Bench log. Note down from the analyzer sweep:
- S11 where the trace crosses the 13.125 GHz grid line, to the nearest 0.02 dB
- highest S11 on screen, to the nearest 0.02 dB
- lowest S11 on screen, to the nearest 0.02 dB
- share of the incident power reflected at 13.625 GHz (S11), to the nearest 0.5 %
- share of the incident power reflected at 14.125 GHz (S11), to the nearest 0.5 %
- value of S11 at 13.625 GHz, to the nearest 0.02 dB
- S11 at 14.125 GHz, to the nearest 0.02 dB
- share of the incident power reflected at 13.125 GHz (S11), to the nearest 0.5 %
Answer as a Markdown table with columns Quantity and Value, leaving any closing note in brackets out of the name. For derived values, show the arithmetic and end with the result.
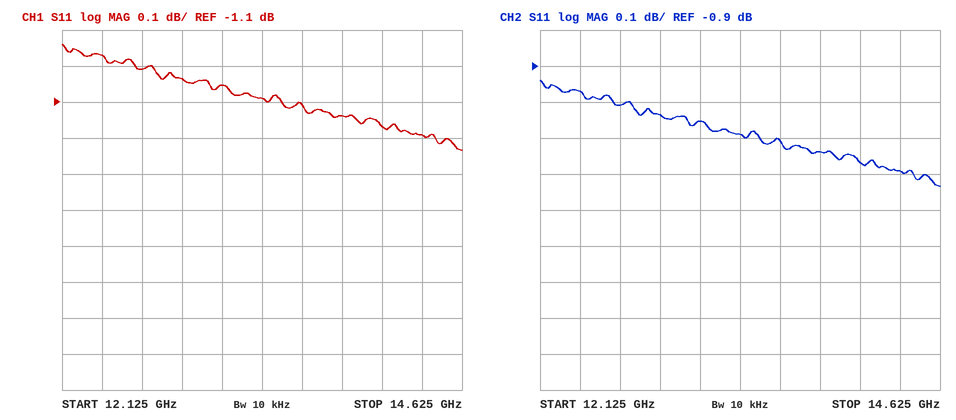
| Quantity | Value |
|---|---|
| S11 where the trace crosses the 13.125 GHz grid line, to the nearest 0.02 dB | -1.06 dB |
| highest S11 on screen, to the nearest 0.02 dB | -0.94 dB |
| lowest S11 on screen, to the nearest 0.02 dB | -1.24 dB |
| share of the incident power reflected at 13.625 GHz (S11), to the nearest 0.5 % | 10^(-1.1/10) ≈ 77.6 %, so 77.5 % to the nearest 0.5 % |
| share of the incident power reflected at 14.125 GHz (S11), to the nearest 0.5 % | 10^(-1.16/10) ≈ 76.6 %, so 76.5 % to the nearest 0.5 % |
| value of S11 at 13.625 GHz, to the nearest 0.02 dB | -1.10 dB |
| S11 at 14.125 GHz, to the nearest 0.02 dB | -1.16 dB |
| share of the incident power reflected at 13.125 GHz (S11), to the nearest 0.5 % | 10^(-1.06/10) ≈ 78.3 %, so 78.5 % to the nearest 0.5 % |
